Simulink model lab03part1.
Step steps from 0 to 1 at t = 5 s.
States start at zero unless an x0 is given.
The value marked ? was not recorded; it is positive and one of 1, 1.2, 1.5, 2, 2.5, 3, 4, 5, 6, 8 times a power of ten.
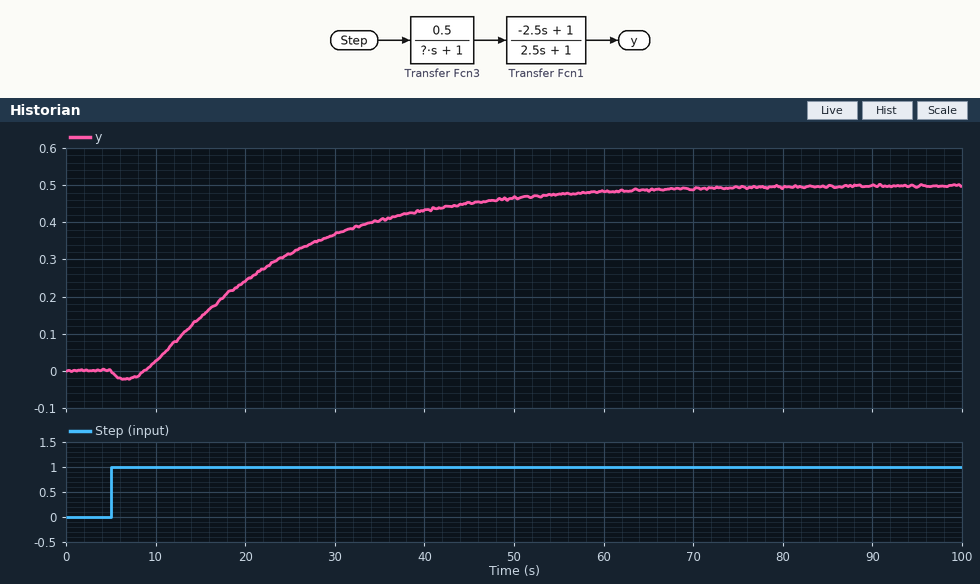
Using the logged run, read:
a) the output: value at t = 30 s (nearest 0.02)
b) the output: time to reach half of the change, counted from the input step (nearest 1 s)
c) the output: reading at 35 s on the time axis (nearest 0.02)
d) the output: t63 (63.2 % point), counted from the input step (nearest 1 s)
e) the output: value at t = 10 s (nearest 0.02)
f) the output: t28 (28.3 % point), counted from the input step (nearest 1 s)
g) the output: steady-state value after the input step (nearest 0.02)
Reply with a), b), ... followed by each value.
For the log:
a) 0.36
b) 15 s
c) 0.40
d) 20 s
e) 0.02
f) 10 s
g) 0.50
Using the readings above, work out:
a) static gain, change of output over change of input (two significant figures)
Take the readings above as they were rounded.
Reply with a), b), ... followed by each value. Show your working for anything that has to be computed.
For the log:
a) (0.5 - 0) / (1 - 0) = 0.50
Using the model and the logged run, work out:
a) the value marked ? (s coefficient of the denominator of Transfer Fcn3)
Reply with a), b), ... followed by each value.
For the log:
a) 15
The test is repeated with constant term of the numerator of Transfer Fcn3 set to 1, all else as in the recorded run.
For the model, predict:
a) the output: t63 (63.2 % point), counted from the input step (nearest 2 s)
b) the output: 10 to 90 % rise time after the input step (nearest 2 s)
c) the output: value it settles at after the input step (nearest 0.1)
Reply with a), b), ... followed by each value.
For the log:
a) 20 s
b) 34 s
c) 1.0
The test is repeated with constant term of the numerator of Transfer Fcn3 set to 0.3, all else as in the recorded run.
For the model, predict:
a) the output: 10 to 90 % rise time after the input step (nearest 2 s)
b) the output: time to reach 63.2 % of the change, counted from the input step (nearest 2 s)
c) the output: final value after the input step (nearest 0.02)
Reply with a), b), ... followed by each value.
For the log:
a) 34 s
b) 20 s
c) 0.30
